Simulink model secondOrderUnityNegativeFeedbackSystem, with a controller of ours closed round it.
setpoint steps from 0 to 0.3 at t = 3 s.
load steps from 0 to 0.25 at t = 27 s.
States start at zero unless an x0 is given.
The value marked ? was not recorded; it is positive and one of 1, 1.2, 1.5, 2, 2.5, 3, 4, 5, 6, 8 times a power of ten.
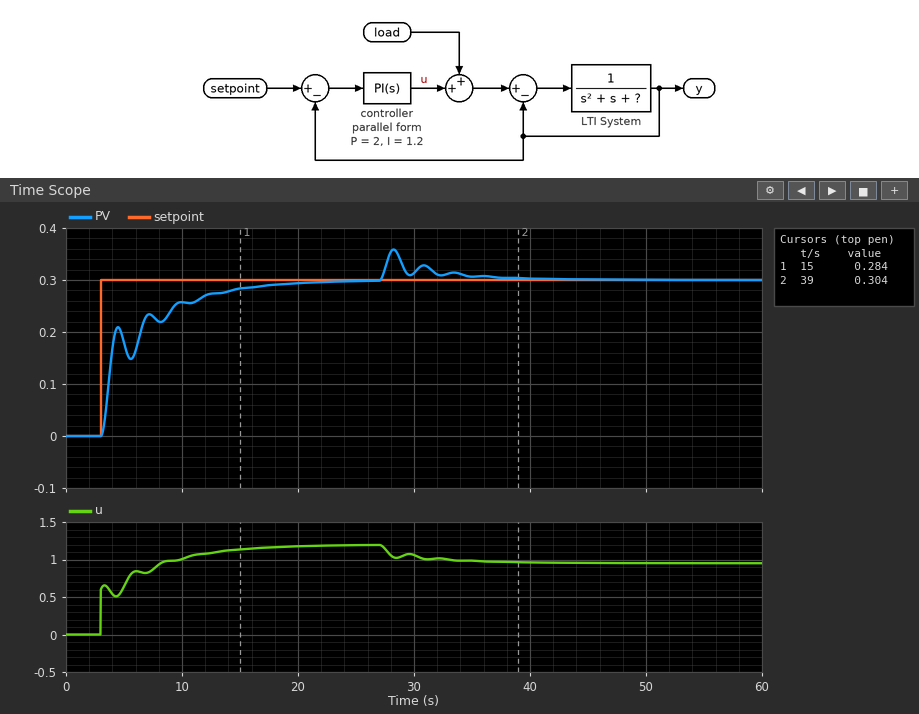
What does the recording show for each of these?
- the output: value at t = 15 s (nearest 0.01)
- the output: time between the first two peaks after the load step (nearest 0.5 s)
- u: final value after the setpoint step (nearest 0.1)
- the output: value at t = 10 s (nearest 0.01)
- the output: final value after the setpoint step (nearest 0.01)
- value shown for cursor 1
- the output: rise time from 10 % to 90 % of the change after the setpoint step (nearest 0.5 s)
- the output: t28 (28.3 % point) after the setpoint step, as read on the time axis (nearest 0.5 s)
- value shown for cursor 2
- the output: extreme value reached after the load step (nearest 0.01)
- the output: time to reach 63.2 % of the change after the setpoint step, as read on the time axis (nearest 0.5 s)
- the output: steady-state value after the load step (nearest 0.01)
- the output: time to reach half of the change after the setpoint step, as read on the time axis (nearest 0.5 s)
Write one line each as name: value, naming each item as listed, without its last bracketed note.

the output: value at t = 15 s: 0.28
the output: time between the first two peaks after the load step: 2.5 s
u: final value after the setpoint step: 1.2
the output: value at t = 10 s: 0.26
the output: final value after the setpoint step: 0.30
value shown for cursor 1: 0.284
the output: rise time from 10 % to 90 % of the change after the setpoint step: 8.5 s
the output: t28 (28.3 % point) after the setpoint step, as read on the time axis: 3.5 s
value shown for cursor 2: 0.304
the output: extreme value reached after the load step: 0.36
the output: time to reach 63.2 % of the change after the setpoint step, as read on the time axis: 4.0 s
the output: steady-state value after the load step: 0.30
the output: time to reach half of the change after the setpoint step, as read on the time axis: 4.0 s
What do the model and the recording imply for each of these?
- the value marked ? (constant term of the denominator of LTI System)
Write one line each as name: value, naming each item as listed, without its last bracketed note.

the value marked ?: 3
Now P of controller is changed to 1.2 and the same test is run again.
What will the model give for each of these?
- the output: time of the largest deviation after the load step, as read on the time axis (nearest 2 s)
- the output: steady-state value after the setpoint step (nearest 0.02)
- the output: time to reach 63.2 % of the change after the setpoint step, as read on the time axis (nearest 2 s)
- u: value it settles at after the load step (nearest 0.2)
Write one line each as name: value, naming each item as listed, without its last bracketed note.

the output: time of the largest deviation after the load step, as read on the time axis: 28 s
the output: steady-state value after the setpoint step: 0.30
the output: time to reach 63.2 % of the change after the setpoint step, as read on the time axis: 6 s
u: value it settles at after the load step: 1.0
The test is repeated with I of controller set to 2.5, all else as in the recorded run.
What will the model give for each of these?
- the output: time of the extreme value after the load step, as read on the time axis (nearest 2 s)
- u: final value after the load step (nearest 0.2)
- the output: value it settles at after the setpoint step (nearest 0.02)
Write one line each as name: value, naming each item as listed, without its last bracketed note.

the output: time of the extreme value after the load step, as read on the time axis: 28 s
u: final value after the load step: 1.0
the output: value it settles at after the setpoint step: 0.30
